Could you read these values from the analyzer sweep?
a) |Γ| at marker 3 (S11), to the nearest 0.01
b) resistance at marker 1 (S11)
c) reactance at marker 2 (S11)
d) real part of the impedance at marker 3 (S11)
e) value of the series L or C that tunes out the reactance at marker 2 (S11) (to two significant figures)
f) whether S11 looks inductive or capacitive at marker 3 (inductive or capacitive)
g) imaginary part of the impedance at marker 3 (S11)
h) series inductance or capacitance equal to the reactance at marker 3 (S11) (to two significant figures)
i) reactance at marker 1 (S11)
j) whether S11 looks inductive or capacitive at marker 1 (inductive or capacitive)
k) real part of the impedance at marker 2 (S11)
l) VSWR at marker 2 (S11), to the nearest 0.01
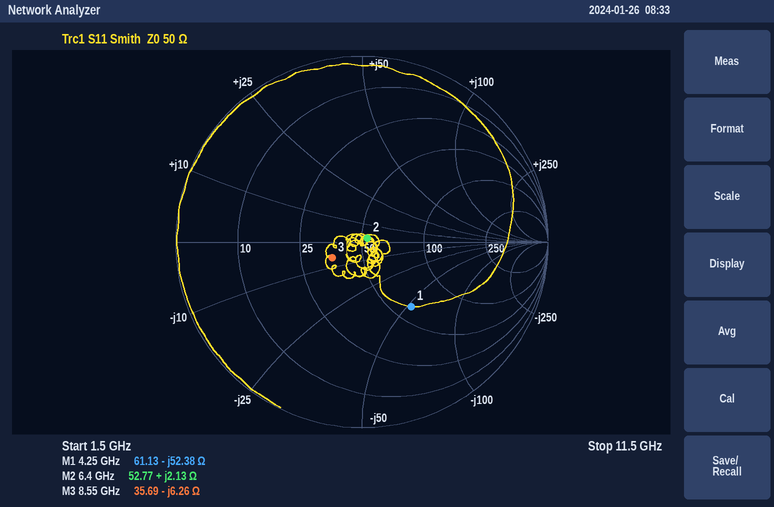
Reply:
0.18
61.13 Ω
+2.13 Ω
35.69 Ω
12 pF
capacitive
-6.26 Ω
3.0 pF
-52.38 Ω
capacitive
52.77 Ω
1.07
